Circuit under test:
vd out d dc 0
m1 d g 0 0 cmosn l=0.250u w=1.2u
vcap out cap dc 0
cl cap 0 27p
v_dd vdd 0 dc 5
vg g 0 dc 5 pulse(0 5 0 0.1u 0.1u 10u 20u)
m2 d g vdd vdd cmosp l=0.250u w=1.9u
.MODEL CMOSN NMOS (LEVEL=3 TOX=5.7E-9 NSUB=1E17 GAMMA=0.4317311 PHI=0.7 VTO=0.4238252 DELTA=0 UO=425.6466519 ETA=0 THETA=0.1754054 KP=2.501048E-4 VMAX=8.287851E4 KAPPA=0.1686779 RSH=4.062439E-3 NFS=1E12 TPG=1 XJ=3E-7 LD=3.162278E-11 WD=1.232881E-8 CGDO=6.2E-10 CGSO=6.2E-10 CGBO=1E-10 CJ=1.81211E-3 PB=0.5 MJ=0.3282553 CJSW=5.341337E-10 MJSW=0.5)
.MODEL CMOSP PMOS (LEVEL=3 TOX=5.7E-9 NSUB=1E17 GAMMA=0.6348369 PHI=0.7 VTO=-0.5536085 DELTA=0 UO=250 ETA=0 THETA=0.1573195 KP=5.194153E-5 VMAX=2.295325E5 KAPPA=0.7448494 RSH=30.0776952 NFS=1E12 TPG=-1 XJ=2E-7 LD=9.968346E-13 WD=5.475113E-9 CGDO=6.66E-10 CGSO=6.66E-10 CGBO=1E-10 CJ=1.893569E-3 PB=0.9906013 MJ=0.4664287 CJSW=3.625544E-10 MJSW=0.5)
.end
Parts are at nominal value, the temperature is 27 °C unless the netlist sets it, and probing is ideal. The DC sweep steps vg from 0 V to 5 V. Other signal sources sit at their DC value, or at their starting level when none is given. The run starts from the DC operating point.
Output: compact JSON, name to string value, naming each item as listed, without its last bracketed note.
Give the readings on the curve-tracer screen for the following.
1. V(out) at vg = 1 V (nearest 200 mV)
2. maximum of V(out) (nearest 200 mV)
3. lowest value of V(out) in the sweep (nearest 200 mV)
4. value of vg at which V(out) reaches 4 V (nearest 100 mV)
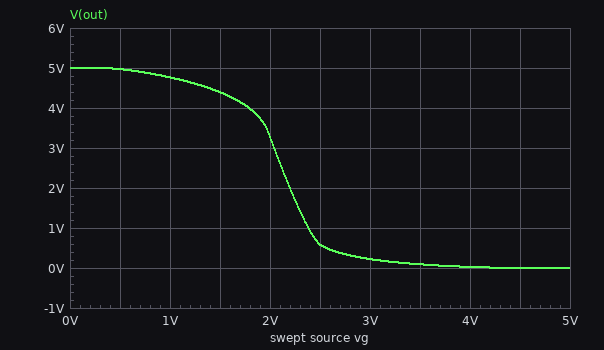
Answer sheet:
{"V(out) at vg = 1 V": "4.8 V", "maximum of V(out)": "5.0 V", "lowest value of V(out) in the sweep": "0 V", "value of vg at which V(out) reaches 4 V": "1.8 V"}
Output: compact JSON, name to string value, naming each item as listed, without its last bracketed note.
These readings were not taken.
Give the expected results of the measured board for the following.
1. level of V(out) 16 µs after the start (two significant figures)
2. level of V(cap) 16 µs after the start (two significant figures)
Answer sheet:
{"level of V(out) 16 µs after the start": "5.0 V", "level of V(cap) 16 µs after the start": "5.0 V"}
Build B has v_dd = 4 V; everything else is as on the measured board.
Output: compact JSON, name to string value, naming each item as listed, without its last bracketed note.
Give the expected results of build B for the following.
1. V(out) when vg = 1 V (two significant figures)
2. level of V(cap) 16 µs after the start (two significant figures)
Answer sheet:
{"V(out) when vg = 1 V": "3.7 V", "level of V(cap) 16 µs after the start": "4.0 V"}
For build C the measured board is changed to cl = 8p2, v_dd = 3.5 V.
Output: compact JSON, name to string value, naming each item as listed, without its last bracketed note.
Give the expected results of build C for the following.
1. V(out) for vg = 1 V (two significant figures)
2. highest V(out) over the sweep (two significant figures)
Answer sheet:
{"V(out) for vg = 1 V": "3.2 V", "highest V(out) over the sweep": "3.5 V"}
